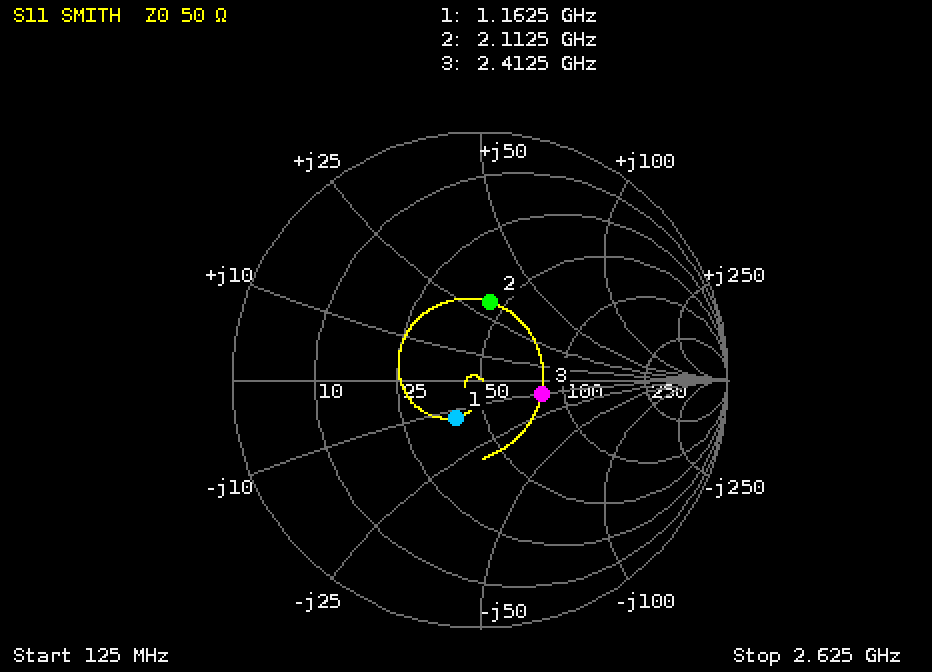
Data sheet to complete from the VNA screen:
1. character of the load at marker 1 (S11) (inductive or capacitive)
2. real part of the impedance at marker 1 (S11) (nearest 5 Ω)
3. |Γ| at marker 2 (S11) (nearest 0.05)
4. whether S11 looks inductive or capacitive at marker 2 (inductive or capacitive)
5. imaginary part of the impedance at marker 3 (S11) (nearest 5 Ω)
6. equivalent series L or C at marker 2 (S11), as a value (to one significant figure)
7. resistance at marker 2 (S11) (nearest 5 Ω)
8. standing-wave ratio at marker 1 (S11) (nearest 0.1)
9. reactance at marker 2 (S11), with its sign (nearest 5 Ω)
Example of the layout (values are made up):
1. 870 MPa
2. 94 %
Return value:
1. capacitive
2. 40 Ω
3. 0.30
4. inductive
5. -10 Ω
6. 2 nH
7. 45 Ω
8. 1.4
9. +30 Ω
